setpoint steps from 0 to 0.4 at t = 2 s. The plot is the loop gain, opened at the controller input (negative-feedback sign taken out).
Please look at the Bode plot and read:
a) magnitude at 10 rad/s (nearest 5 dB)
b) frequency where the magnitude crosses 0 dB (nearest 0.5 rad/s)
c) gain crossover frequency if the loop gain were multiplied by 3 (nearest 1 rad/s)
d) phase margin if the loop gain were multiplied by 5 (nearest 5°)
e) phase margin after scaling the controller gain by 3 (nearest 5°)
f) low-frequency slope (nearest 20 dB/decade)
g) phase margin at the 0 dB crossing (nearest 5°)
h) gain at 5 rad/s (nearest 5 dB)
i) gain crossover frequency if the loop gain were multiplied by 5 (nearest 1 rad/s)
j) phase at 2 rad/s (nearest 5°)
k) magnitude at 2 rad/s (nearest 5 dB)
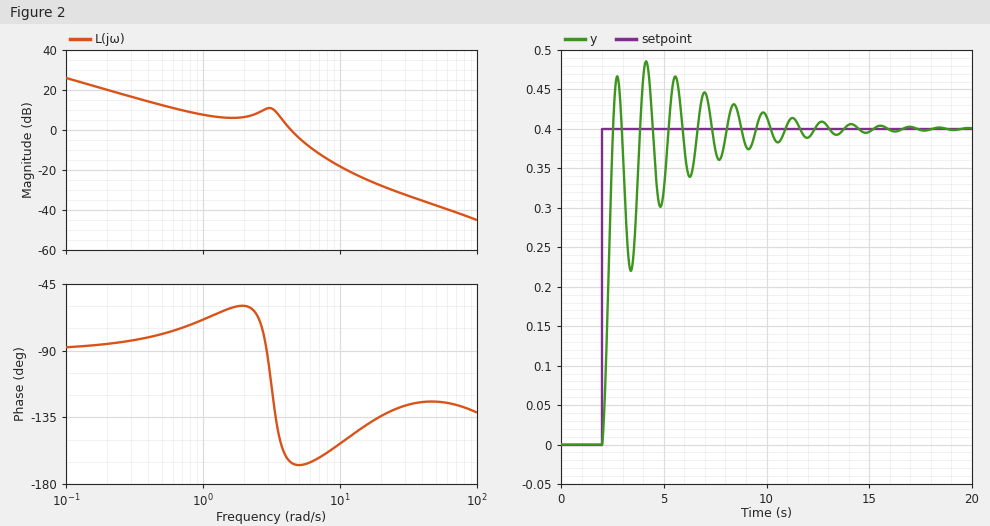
-20 dB
4.5 rad/s
6 rad/s
20°
15°
-20 dB/decade
15°
-5 dB
8 rad/s
-60°
5 dB
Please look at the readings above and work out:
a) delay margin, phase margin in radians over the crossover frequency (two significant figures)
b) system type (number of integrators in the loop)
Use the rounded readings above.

0.058 s
1
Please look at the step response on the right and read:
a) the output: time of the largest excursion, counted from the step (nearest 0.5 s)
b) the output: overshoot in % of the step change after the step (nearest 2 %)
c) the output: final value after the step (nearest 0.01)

2.0 s
22 %
0.40
